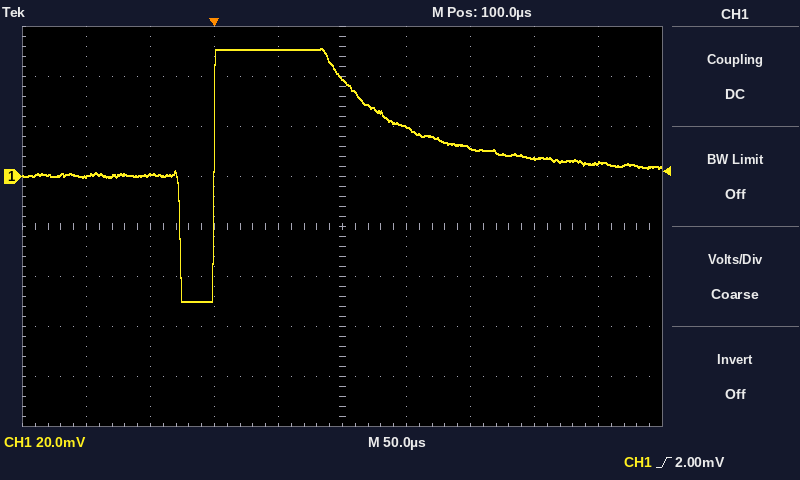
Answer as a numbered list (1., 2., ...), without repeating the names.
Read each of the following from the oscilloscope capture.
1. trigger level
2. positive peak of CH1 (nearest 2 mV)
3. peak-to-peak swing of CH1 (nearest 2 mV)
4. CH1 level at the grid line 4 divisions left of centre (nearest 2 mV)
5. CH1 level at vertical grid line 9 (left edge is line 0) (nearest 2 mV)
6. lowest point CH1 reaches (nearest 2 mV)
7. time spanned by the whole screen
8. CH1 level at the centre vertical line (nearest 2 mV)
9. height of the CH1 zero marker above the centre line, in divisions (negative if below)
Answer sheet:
1. 2.00 mV
2. 52 mV
3. 102 mV
4. 0 mV
5. 6 mV
6. -50 mV
7. 500 µs
8. 40 mV
9. +1.0 div
